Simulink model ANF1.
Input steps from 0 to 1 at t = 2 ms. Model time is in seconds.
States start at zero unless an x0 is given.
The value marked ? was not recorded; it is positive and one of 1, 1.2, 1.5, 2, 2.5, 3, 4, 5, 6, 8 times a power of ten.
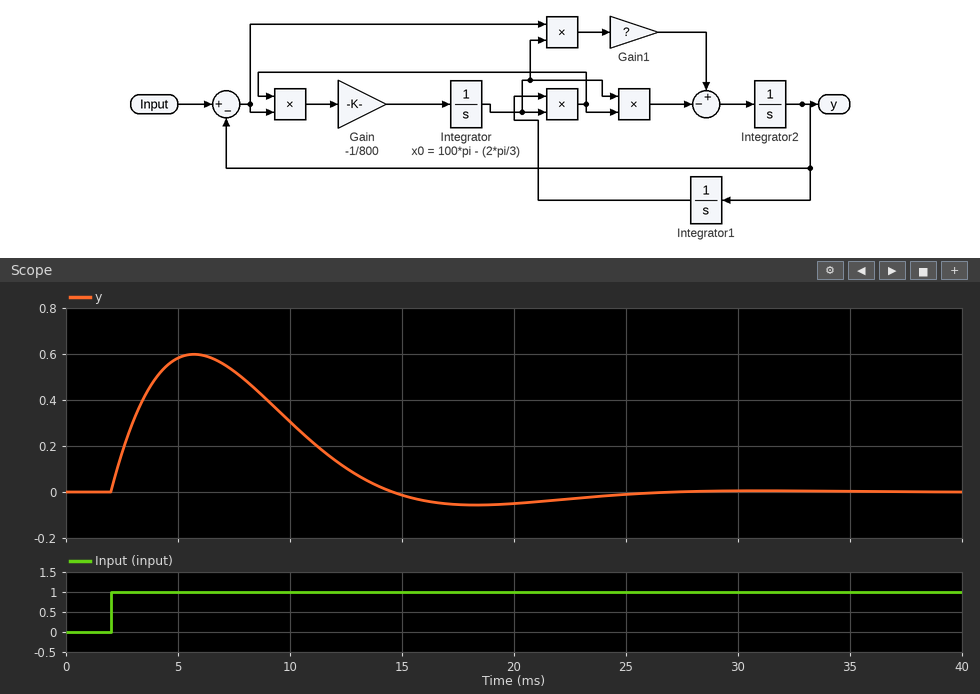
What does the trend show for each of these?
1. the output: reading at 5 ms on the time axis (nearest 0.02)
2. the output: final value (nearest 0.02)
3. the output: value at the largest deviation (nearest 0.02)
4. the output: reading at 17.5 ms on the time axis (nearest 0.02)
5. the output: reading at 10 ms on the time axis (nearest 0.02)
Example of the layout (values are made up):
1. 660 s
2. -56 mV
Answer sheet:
1. 0.58
2. 0.00
3. 0.60
4. -0.06
5. 0.30
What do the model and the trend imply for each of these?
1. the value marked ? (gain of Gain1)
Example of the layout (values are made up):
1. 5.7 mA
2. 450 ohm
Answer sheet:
1. 1.2
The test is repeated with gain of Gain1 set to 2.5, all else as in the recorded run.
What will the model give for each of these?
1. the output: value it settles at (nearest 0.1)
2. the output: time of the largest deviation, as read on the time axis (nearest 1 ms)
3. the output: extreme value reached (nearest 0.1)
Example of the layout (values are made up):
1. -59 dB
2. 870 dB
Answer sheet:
1. 0.0
2. 5 ms
3. 0.8
